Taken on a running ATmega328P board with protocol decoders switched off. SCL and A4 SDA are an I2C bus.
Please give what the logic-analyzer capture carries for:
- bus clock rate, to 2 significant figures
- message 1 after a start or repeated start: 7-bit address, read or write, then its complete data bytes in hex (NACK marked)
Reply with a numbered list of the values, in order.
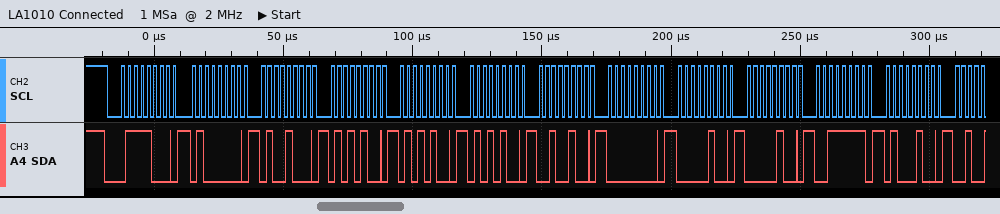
1. 400 kHz
2. 0x3C write: 40 48 54 54 54 24 00 04 04 3F 44
